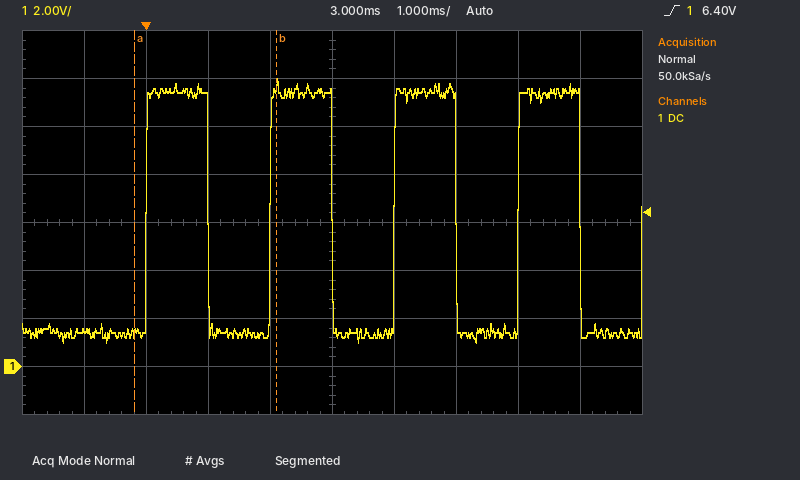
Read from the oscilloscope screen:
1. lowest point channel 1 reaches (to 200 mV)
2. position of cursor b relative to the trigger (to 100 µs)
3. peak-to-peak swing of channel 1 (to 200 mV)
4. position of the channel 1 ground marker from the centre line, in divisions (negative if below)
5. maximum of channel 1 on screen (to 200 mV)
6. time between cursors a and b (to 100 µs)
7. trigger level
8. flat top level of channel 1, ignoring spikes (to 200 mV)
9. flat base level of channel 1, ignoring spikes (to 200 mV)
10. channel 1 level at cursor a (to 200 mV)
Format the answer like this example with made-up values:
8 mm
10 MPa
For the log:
1.0 V
+2.1 ms
11.0 V
-3.0 div
12.0 V
2.3 ms
6.40 V
11.4 V
1.4 V
1.4 V
